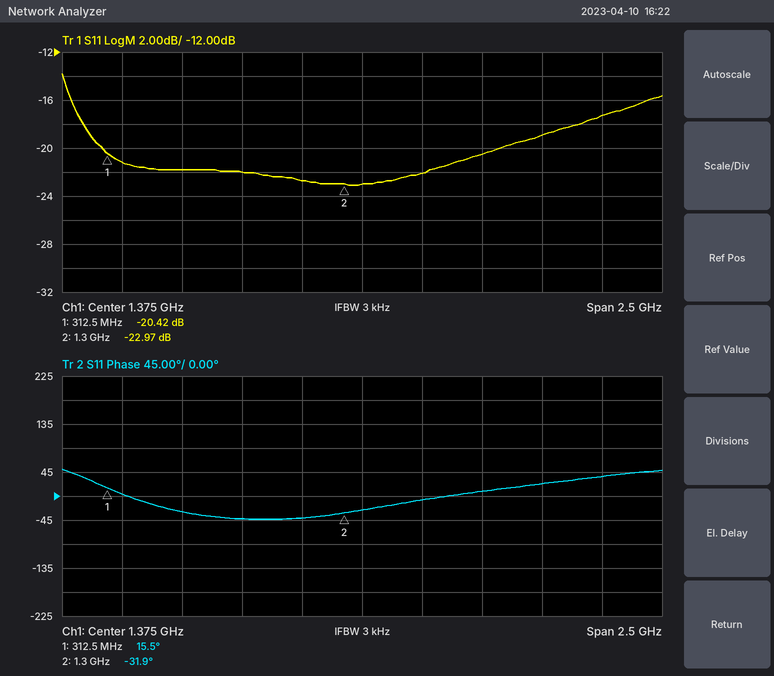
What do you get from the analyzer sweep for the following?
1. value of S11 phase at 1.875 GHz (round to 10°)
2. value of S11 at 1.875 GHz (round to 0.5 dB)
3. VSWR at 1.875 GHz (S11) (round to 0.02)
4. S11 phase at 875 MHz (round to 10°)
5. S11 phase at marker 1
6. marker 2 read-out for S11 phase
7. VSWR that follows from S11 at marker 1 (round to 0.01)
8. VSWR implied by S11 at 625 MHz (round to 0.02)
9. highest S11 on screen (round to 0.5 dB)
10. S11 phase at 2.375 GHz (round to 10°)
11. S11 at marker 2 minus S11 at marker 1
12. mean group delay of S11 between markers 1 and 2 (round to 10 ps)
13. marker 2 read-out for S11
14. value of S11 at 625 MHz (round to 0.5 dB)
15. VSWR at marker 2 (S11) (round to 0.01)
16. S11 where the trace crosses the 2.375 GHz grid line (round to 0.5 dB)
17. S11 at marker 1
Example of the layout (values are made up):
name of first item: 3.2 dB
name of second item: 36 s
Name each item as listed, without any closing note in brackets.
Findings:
value of S11 phase at 1.875 GHz: 10°
value of S11 at 1.875 GHz: -20.5 dB
VSWR at 1.875 GHz (S11): 1.20
S11 phase at 875 MHz: -40°
S11 phase at marker 1: 15.5°
marker 2 read-out for S11 phase: -31.9°
VSWR that follows from S11 at marker 1: 1.21
VSWR implied by S11 at 625 MHz: 1.18
highest S11 on screen: -14.0 dB
S11 phase at 2.375 GHz: 40°
S11 at marker 2 minus S11 at marker 1: -2.55 dB
mean group delay of S11 between markers 1 and 2: 130 ps
marker 2 read-out for S11: -22.97 dB
value of S11 at 625 MHz: -22.0 dB
VSWR at marker 2 (S11): 1.15
S11 where the trace crosses the 2.375 GHz grid line: -17.5 dB
S11 at marker 1: -20.42 dB
